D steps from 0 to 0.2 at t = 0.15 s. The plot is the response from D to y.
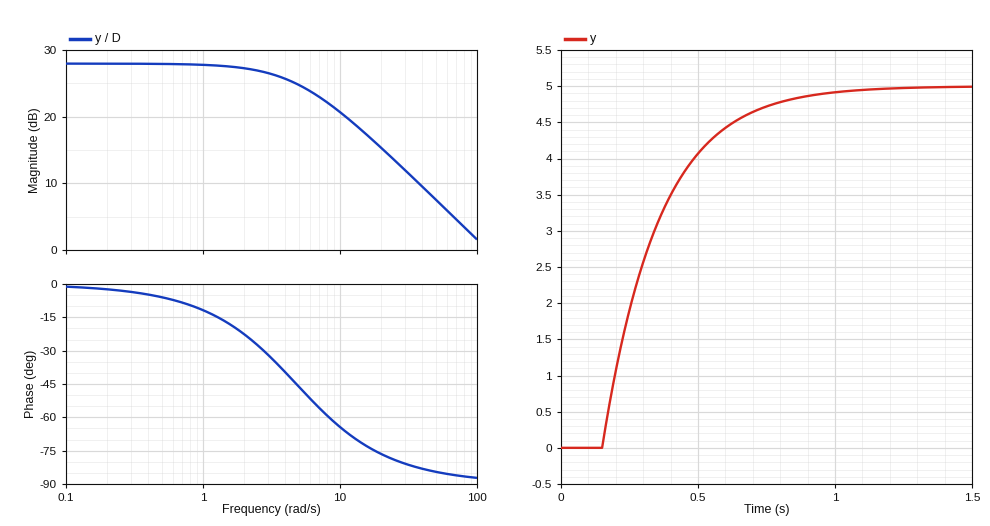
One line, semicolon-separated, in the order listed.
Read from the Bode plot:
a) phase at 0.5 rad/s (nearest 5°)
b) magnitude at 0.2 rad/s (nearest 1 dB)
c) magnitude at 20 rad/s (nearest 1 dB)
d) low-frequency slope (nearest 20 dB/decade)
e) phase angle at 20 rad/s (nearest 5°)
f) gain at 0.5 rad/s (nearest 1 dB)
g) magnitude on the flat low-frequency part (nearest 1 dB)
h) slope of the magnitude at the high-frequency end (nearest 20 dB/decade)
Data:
-5°; 28 dB; 15 dB; 0 dB/decade; -75°; 28 dB; 28 dB; -20 dB/decade
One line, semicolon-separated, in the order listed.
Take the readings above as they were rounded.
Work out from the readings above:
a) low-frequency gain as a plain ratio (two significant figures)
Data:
25
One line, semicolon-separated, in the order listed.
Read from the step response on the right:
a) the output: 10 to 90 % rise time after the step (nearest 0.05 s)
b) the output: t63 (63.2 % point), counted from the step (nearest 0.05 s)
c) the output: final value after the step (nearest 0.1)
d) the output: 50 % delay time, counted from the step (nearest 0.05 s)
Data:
0.45 s; 0.20 s; 5.0; 0.15 s
